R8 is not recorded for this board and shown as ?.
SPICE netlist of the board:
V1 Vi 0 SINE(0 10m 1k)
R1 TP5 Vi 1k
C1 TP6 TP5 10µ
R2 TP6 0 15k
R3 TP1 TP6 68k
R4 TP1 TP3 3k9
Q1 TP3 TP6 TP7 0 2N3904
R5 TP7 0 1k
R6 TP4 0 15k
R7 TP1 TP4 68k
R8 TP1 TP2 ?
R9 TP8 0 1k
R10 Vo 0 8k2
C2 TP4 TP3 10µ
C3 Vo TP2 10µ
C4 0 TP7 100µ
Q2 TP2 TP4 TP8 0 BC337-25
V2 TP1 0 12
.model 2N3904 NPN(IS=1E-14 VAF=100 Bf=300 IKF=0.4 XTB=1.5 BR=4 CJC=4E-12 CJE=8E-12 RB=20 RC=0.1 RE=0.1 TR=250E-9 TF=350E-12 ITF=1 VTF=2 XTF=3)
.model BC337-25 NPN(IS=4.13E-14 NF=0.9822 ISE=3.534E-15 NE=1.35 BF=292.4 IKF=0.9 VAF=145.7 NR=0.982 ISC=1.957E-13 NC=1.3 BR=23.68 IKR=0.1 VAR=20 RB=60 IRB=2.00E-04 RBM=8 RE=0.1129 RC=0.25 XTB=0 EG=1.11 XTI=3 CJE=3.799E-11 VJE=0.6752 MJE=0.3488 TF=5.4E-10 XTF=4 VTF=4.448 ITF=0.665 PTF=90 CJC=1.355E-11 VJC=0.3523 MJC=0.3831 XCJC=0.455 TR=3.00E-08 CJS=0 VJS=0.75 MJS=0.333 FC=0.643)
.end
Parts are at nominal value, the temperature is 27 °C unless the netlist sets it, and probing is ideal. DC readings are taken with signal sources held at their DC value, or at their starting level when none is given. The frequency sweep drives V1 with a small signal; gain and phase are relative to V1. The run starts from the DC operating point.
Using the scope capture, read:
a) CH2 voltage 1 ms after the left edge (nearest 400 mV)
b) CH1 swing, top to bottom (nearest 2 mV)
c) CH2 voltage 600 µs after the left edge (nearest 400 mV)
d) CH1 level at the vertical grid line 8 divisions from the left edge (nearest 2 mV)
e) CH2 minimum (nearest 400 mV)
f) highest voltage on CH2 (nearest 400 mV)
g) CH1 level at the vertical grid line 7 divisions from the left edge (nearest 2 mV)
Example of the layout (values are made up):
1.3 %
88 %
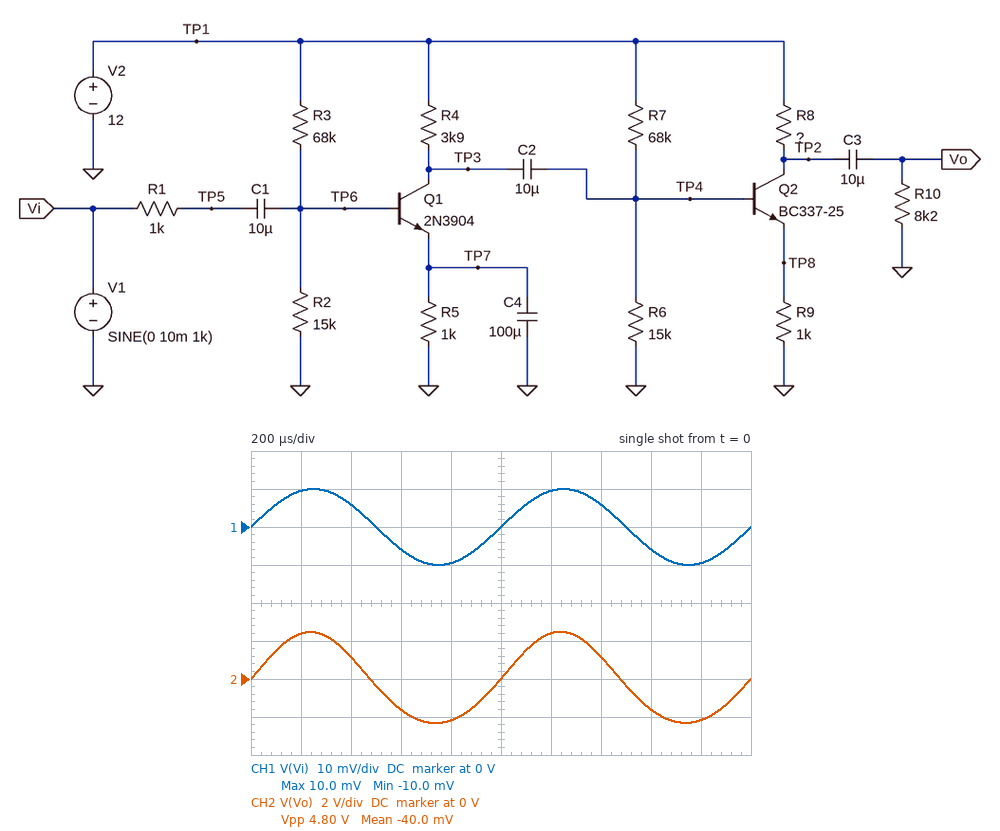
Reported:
0 V
20 mV
-1.6 V
-6 mV
-2.4 V
2.4 V
6 mV
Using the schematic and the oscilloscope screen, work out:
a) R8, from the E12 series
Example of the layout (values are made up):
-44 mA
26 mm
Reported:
2.7 kΩ
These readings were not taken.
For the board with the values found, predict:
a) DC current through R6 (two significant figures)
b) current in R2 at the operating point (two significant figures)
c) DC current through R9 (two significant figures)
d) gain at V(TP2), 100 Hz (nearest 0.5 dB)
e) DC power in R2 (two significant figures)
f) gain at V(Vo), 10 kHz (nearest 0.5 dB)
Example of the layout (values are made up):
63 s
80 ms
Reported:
140 µA
140 µA
1.5 mA
46.0 dB
300 µW
48.0 dB
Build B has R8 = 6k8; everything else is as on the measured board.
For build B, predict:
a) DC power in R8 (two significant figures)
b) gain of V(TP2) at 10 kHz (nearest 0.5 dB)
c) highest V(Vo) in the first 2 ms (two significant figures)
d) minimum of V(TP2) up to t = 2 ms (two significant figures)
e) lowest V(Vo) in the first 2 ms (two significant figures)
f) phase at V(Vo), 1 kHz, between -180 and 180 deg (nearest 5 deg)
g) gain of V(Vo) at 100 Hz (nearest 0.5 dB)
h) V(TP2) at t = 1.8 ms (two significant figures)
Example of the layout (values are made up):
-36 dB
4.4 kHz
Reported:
15 mW
53.0 dB
4.6 V
1.6 V
-340 mV
5 deg
51.0 dB
1.8 V
